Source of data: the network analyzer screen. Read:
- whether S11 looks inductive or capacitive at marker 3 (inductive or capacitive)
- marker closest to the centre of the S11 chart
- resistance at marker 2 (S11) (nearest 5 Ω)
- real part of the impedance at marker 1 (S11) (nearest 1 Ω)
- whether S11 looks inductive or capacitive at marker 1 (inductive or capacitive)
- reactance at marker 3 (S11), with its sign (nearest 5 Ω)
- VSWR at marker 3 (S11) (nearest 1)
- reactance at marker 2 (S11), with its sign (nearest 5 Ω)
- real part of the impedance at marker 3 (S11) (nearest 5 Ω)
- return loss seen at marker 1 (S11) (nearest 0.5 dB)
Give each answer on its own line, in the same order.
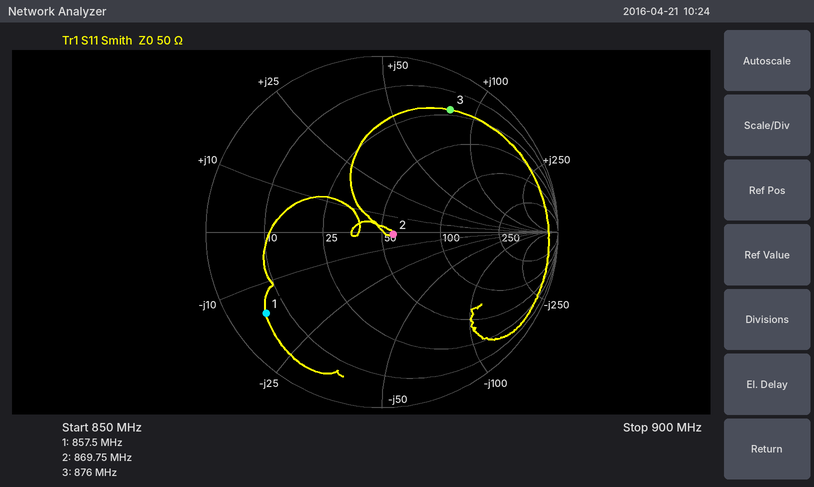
inductive
marker 2
55 Ω
6 Ω
capacitive
+80 Ω
9
0 Ω
20 Ω
2.0 dB
